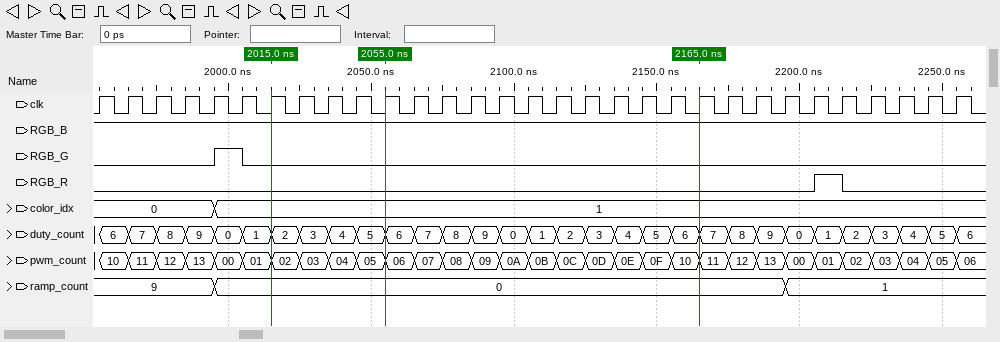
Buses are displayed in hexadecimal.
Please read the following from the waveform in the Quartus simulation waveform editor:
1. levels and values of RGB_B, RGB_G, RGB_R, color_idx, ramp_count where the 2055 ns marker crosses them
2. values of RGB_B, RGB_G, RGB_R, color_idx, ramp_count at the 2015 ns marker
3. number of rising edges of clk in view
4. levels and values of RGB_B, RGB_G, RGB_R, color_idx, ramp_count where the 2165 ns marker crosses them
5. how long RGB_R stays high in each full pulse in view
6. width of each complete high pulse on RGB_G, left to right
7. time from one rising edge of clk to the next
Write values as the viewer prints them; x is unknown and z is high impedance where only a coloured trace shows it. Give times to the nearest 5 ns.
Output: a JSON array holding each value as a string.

["RGB_B=1, RGB_G=0, RGB_R=0, color_idx=1, ramp_count=0", "RGB_B=1, RGB_G=0, RGB_R=0, color_idx=1, ramp_count=0", "31", "RGB_B=1, RGB_G=0, RGB_R=0, color_idx=1, ramp_count=0", "10 ns", "10 ns", "10 ns"]
